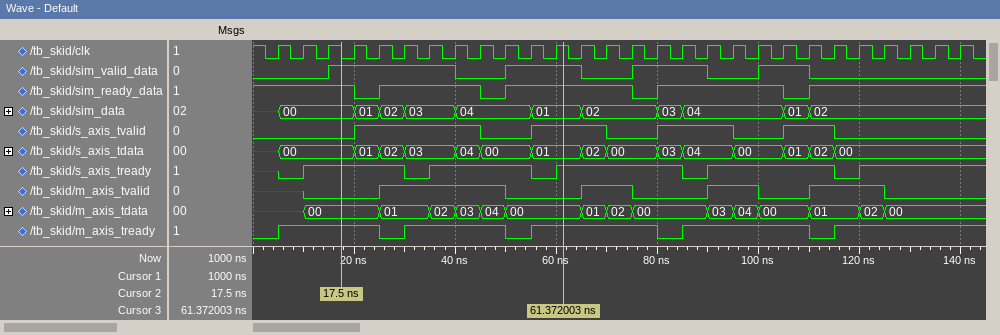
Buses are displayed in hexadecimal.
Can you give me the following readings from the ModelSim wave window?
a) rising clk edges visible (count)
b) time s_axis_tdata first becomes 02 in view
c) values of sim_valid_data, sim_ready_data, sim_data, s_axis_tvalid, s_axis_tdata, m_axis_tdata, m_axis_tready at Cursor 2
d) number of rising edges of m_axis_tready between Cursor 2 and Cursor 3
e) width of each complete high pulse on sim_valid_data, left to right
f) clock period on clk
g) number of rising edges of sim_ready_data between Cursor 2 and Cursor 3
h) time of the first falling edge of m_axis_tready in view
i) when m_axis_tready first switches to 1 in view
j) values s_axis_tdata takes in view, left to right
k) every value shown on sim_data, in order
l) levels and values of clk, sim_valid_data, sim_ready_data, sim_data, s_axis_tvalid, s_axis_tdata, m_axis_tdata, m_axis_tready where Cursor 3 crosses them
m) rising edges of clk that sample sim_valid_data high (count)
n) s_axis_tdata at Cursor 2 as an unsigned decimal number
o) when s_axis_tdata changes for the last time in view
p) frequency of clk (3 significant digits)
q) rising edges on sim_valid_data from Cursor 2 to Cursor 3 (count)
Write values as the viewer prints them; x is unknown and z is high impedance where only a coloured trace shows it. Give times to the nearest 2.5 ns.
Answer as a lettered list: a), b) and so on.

a) 28
b) 25 ns
c) sim_valid_data=1, sim_ready_data=1, sim_data=00, s_axis_tvalid=0, s_axis_tdata=00, m_axis_tdata=00, m_axis_tready=1
d) 2
e) 25 ns, 15 ns, 15 ns, 10 ns
f) 5 ns
g) 2
h) 25 ns
i) 5 ns
j) x, 00, 01, 02, 03, 04, 00, 01, 02, 00, 03, 04, 00, 01, 02, 00
k) x, 00, 01, 02, 03, 04, 01, 02, 03, 04, 01, 02
l) clk=1, sim_valid_data=1, sim_ready_data=1, sim_data=01, s_axis_tvalid=1, s_axis_tdata=01, m_axis_tdata=00, m_axis_tready=1
m) 13
n) 0
o) 115 ns
p) 200 MHz
q) 1
